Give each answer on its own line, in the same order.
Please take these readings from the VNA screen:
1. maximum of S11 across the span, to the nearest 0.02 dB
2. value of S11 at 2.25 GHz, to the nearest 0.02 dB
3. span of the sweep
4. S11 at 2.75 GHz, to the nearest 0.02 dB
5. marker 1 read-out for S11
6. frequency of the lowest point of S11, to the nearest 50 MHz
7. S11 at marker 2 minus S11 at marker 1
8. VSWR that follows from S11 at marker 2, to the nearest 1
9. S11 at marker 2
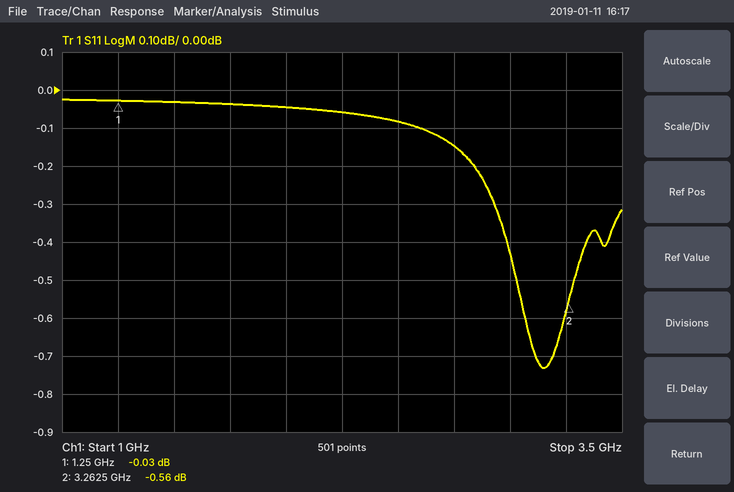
-0.02 dB
-0.06 dB
2.5 GHz
-0.14 dB
-0.03 dB
3.15 GHz
-0.53 dB
31
-0.56 dB
